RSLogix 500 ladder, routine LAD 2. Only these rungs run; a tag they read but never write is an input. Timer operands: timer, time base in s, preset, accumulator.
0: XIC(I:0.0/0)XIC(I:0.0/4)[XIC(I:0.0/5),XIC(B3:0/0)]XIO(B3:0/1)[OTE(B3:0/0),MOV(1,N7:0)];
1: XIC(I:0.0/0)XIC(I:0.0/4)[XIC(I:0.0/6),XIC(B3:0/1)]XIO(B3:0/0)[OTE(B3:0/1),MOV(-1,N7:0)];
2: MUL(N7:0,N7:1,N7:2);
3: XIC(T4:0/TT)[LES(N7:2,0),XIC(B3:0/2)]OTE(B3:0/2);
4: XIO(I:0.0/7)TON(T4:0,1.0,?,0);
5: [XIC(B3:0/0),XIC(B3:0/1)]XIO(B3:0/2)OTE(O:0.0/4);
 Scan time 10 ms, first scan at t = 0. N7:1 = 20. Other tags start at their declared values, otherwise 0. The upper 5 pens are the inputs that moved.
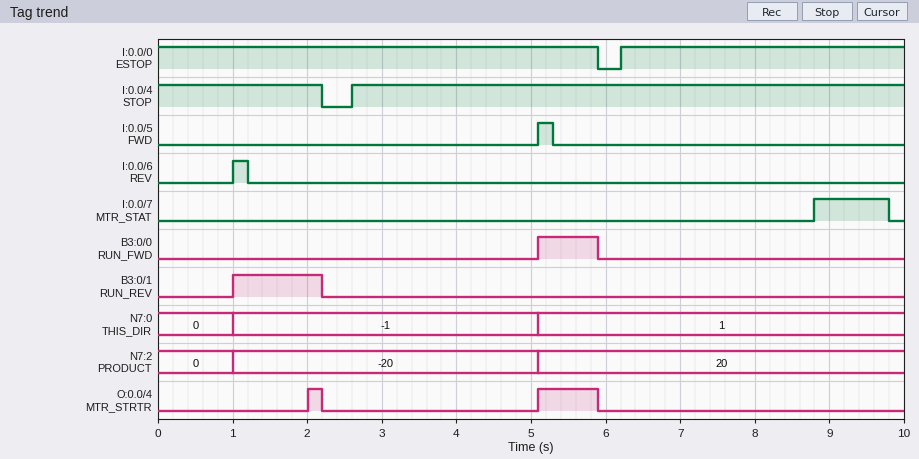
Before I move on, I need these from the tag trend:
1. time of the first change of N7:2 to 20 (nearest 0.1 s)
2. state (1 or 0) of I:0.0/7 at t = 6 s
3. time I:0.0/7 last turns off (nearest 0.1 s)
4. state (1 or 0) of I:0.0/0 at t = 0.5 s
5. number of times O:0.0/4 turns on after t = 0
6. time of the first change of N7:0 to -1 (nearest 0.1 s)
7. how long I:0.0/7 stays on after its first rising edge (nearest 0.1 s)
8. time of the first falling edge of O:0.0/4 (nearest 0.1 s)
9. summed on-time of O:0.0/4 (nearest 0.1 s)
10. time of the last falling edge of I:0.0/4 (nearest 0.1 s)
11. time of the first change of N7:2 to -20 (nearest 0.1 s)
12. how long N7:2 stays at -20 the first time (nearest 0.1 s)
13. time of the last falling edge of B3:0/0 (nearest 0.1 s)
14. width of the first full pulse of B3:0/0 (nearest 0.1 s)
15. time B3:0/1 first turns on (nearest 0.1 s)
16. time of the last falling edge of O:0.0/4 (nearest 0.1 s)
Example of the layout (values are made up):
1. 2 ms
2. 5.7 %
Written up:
1. 5.1 s
2. 0
3. 9.8 s
4. 1
5. 2
6. 1.0 s
7. 1.0 s
8. 2.2 s
9. 1.0 s
10. 2.2 s
11. 1.0 s
12. 4.1 s
13. 5.9 s
14. 0.8 s
15. 1.0 s
16. 5.9 s
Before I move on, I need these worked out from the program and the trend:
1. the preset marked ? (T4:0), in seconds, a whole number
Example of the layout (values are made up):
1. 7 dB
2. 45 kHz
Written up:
1. 2 s
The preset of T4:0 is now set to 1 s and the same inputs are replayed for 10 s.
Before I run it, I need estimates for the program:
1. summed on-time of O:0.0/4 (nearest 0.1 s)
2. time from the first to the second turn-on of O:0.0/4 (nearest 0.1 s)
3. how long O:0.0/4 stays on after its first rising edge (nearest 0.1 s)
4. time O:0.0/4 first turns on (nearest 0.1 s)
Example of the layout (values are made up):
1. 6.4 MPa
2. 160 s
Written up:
1. 2.0 s
2. 4.1 s
3. 1.2 s
4. 1.0 s
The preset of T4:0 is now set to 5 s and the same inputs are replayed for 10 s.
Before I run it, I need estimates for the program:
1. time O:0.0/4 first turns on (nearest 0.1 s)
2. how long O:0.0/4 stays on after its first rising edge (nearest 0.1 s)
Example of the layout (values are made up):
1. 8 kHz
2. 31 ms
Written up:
1. 5.1 s
2. 0.8 s
